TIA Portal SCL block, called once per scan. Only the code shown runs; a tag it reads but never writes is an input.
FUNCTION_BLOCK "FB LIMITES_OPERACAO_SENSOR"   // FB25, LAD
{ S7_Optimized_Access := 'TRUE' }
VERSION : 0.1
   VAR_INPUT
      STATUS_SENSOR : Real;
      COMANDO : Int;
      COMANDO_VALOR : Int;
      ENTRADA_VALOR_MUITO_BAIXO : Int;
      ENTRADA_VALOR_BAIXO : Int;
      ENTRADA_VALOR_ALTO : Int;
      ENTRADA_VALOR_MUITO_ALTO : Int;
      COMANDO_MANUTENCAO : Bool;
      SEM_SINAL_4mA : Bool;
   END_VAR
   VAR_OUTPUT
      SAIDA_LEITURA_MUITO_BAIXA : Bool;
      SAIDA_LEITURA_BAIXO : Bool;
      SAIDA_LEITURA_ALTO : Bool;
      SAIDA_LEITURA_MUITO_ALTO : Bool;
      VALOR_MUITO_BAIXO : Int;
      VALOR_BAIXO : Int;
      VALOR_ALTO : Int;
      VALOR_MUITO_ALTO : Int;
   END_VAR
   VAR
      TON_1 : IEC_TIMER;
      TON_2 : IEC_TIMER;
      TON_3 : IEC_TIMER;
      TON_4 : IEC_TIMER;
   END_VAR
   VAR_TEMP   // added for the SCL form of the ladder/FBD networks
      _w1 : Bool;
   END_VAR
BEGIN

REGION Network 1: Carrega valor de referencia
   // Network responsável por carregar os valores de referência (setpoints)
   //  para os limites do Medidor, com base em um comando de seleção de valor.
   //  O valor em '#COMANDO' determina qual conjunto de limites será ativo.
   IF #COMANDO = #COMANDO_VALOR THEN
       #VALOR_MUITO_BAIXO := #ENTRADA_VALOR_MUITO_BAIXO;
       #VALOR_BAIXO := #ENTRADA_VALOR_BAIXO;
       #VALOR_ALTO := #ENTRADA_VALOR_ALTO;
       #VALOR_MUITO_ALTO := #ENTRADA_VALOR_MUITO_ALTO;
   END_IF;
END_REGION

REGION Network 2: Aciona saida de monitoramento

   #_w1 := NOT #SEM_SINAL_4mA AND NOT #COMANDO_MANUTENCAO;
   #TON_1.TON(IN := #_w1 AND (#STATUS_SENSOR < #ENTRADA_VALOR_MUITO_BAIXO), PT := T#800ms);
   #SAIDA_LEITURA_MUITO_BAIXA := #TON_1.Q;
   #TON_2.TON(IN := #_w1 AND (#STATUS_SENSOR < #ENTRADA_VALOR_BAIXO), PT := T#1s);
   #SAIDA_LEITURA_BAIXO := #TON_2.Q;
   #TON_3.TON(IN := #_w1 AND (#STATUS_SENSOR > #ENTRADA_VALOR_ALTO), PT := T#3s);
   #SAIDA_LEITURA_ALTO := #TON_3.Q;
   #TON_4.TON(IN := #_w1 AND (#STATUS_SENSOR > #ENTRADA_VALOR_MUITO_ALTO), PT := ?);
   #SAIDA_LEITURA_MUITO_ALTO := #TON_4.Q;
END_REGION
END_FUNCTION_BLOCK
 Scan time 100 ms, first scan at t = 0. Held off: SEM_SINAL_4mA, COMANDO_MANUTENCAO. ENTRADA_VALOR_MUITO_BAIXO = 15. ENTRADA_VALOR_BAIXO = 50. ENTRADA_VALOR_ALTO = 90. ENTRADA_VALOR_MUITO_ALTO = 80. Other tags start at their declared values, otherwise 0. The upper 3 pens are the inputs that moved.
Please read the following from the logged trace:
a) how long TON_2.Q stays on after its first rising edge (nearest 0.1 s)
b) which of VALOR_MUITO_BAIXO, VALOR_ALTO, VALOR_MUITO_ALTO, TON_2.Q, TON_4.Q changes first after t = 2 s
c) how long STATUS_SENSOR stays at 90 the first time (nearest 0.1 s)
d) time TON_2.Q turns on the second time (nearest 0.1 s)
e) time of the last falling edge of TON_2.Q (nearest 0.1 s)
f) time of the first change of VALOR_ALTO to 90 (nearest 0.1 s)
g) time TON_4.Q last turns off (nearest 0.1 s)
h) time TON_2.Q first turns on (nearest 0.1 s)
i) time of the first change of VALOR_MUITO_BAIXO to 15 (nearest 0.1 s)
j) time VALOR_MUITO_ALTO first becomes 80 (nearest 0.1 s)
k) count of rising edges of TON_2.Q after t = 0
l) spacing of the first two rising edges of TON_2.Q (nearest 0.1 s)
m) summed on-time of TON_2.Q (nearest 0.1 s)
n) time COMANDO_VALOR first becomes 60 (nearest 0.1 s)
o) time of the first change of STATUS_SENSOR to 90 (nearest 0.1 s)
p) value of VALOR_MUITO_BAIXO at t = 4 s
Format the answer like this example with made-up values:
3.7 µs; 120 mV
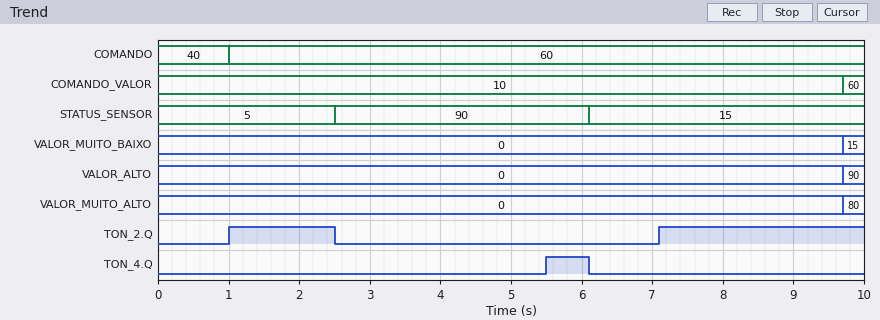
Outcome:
1.5 s; TON_2.Q; 3.6 s; 7.1 s; 2.5 s; 9.7 s; 6.1 s; 1.0 s; 9.7 s; 9.7 s; 2; 6.1 s; 4.4 s; 9.7 s; 2.5 s; 0
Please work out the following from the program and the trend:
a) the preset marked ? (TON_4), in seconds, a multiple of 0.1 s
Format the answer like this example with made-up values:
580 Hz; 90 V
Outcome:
3.0 s
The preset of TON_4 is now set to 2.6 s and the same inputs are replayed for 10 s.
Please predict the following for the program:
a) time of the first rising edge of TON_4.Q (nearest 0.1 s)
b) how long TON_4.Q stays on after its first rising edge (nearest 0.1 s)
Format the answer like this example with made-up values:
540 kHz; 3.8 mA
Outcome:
5.1 s; 1.0 s
